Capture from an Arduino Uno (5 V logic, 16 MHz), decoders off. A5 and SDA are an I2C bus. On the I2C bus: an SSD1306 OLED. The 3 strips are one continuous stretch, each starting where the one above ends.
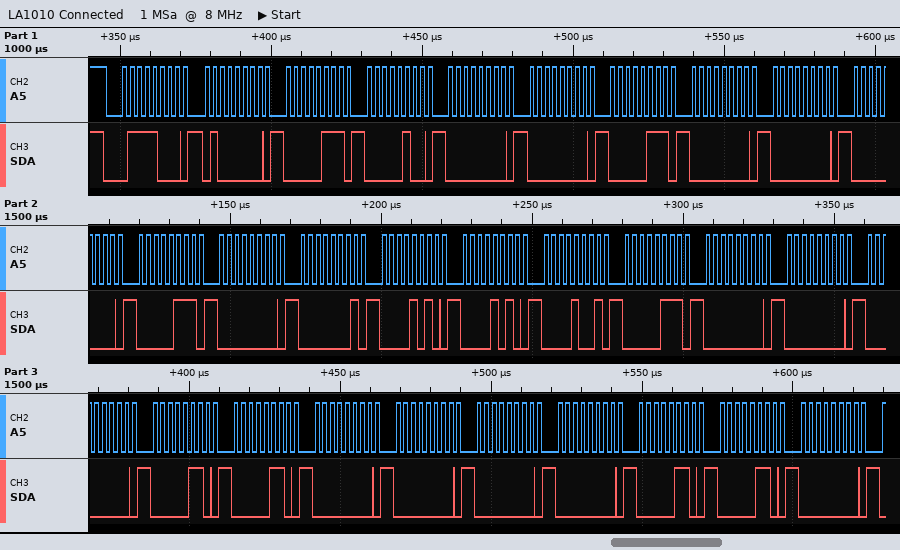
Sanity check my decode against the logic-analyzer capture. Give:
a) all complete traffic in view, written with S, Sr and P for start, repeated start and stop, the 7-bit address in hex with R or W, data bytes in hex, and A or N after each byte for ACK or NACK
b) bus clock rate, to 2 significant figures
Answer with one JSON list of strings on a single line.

["S 3CW A 40 A 07 A 04 A 00 A 00 A 07 A 00 A 00 A 00 A 07 A 00 A 01 A 0A A 0A A 09 A 07 A 00 A 00 A 00 A 06 A 06 A 00 A 00 A 00 A 00 A 06 A 06 A 00 A", "400 kHz"]
